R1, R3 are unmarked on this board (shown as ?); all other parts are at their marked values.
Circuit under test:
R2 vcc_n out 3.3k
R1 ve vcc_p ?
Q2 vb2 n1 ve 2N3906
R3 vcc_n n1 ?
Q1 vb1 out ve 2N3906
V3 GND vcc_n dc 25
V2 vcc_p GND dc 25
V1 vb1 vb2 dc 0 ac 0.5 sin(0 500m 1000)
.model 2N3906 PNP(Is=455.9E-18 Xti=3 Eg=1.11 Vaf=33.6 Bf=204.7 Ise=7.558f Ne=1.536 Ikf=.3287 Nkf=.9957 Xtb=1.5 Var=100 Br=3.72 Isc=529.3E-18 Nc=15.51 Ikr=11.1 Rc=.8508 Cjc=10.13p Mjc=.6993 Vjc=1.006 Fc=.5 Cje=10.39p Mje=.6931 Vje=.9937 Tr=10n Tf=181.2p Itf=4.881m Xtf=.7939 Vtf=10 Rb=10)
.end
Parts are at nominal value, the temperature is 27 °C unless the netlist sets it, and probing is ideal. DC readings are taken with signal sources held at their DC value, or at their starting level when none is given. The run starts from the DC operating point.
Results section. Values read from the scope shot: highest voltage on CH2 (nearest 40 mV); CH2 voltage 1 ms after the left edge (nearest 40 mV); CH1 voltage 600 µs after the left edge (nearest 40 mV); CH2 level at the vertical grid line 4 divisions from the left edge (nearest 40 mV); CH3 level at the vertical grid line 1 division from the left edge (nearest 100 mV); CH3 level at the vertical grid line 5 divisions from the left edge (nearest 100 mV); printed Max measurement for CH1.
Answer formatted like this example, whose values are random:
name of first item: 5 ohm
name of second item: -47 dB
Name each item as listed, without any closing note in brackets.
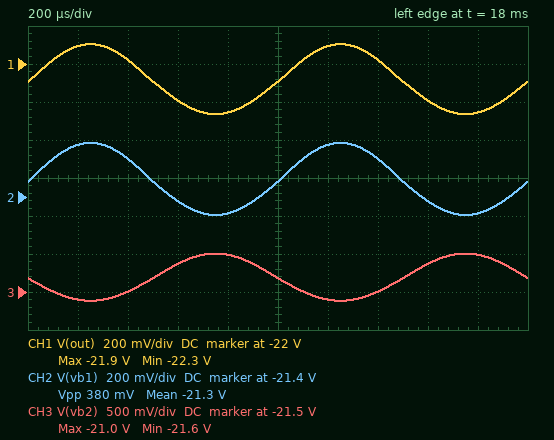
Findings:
highest voltage on CH2: -21.12 V
CH2 voltage 1 ms after the left edge: -21.32 V
CH1 voltage 600 µs after the left edge: -22.20 V
CH2 level at the vertical grid line 4 divisions from the left edge: -21.48 V
CH3 level at the vertical grid line 1 division from the left edge: -21.6 V
CH3 level at the vertical grid line 5 divisions from the left edge: -21.3 V
printed Max measurement for CH1: -21.9 V
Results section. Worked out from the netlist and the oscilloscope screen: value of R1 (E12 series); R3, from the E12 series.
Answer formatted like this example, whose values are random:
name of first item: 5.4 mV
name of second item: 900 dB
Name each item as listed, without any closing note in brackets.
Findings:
value of R1: 33 kΩ
R3, from the E12 series: 5.6 kΩ
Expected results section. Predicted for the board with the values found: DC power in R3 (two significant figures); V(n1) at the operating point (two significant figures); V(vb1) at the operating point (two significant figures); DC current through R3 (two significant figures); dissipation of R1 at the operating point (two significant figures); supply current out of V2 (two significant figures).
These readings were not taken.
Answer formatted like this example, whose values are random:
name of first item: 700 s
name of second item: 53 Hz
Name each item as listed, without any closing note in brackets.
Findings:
DC power in R3: 1.5 mW
V(n1) at the operating point: -22 V
V(vb1) at the operating point: -21 V
DC current through R3: 520 µA
dissipation of R1 at the operating point: 65 mW
supply current out of V2: 1.4 mA
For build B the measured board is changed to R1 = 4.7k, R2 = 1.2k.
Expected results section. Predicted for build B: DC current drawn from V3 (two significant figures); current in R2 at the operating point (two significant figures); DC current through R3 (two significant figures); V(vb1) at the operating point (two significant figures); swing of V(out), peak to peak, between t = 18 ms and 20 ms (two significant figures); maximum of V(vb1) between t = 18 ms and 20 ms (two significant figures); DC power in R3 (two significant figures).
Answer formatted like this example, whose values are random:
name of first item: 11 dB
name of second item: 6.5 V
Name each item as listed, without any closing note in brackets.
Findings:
DC current drawn from V3: 8.6 mA
current in R2 at the operating point: 7.1 mA
DC current through R3: 1.5 mA
V(vb1) at the operating point: -16 V
swing of V(out), peak to peak, between t = 18 ms and 20 ms: 200 mV
maximum of V(vb1) between t = 18 ms and 20 ms: -15 V
DC power in R3: 13 mW
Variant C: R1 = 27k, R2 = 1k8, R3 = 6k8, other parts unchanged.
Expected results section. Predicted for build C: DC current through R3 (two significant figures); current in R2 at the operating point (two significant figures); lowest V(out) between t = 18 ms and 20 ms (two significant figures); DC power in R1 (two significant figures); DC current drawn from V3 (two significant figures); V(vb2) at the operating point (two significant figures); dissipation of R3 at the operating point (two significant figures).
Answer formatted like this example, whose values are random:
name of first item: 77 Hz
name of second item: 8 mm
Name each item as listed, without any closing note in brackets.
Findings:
DC current through R3: 370 µA
current in R2 at the operating point: 1.4 mA
lowest V(out) between t = 18 ms and 20 ms: -23 V
DC power in R1: 81 mW
DC current drawn from V3: 1.7 mA
V(vb2) at the operating point: -22 V
dissipation of R3 at the operating point: 920 µW
